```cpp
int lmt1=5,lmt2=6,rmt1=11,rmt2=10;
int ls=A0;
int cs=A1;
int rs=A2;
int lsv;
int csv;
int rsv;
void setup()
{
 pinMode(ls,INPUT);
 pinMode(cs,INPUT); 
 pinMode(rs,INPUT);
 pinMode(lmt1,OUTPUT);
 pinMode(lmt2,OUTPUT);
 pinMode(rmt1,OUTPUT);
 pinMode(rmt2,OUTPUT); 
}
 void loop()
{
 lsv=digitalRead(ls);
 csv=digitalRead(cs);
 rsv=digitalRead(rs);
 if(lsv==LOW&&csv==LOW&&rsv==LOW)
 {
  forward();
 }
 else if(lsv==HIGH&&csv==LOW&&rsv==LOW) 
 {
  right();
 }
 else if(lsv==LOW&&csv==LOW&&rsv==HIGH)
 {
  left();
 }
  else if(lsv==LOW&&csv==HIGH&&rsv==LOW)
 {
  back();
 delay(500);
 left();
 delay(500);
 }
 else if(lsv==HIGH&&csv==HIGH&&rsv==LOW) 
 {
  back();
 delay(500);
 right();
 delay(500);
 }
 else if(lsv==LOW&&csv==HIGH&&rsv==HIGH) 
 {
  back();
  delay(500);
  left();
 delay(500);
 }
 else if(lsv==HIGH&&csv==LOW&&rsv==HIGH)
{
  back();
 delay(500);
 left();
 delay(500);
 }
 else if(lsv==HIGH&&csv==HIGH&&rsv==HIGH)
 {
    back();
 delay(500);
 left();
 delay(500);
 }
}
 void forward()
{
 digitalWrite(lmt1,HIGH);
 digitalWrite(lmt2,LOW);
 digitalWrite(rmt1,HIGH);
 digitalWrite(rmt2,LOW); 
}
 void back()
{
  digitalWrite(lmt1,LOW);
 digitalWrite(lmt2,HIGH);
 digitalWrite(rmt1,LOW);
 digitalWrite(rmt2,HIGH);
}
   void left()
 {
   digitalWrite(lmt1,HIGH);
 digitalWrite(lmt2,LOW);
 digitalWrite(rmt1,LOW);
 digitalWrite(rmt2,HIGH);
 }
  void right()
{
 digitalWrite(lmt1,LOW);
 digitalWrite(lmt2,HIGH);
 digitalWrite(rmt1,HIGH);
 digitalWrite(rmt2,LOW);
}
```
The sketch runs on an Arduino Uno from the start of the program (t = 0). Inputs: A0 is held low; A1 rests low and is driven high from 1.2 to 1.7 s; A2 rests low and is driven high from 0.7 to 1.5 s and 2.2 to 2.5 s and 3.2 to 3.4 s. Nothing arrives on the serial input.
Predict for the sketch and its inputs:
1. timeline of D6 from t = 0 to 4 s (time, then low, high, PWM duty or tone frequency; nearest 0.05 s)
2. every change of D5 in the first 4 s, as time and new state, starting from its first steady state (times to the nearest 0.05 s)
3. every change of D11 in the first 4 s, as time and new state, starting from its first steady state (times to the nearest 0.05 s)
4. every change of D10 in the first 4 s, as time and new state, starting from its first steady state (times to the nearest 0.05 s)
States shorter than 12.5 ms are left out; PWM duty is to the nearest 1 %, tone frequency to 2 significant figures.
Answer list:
0 s low; 1.2 s high; 1.7 s low
0 s high; 1.2 s low; 1.7 s high
0 s high; 0.7 s low; 2.5 s high; 3.2 s low; 3.4 s high
0 s low; 0.7 s high; 2.5 s low; 3.2 s high; 3.4 s low
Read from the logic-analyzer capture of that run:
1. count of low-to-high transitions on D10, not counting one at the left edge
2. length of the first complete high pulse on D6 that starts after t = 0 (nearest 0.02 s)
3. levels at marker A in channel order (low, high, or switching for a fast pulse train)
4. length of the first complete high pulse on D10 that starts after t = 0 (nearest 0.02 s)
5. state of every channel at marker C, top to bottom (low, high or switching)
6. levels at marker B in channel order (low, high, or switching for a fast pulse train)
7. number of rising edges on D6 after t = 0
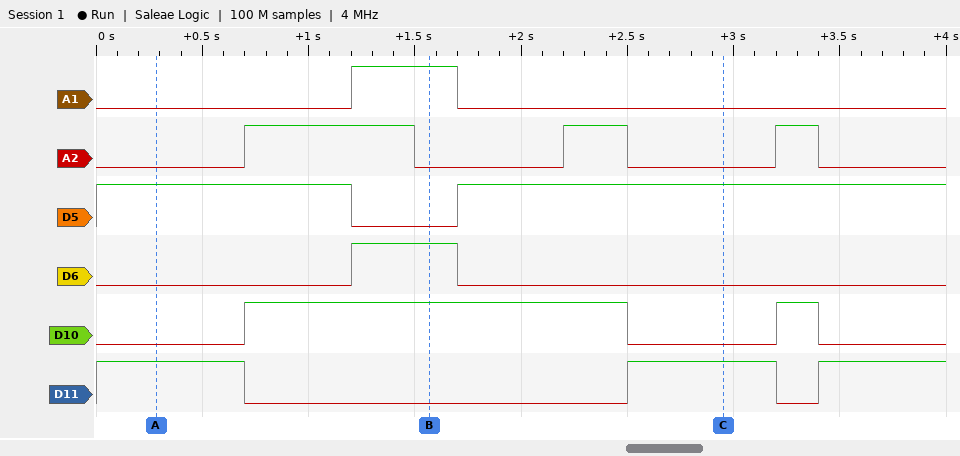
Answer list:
2
0.50 s
A1 low, A2 low, D5 high, D6 low, D10 low, D11 high
1.80 s
A1 low, A2 low, D5 high, D6 low, D10 low, D11 high
A1 high, A2 low, D5 low, D6 high, D10 high, D11 low
1
